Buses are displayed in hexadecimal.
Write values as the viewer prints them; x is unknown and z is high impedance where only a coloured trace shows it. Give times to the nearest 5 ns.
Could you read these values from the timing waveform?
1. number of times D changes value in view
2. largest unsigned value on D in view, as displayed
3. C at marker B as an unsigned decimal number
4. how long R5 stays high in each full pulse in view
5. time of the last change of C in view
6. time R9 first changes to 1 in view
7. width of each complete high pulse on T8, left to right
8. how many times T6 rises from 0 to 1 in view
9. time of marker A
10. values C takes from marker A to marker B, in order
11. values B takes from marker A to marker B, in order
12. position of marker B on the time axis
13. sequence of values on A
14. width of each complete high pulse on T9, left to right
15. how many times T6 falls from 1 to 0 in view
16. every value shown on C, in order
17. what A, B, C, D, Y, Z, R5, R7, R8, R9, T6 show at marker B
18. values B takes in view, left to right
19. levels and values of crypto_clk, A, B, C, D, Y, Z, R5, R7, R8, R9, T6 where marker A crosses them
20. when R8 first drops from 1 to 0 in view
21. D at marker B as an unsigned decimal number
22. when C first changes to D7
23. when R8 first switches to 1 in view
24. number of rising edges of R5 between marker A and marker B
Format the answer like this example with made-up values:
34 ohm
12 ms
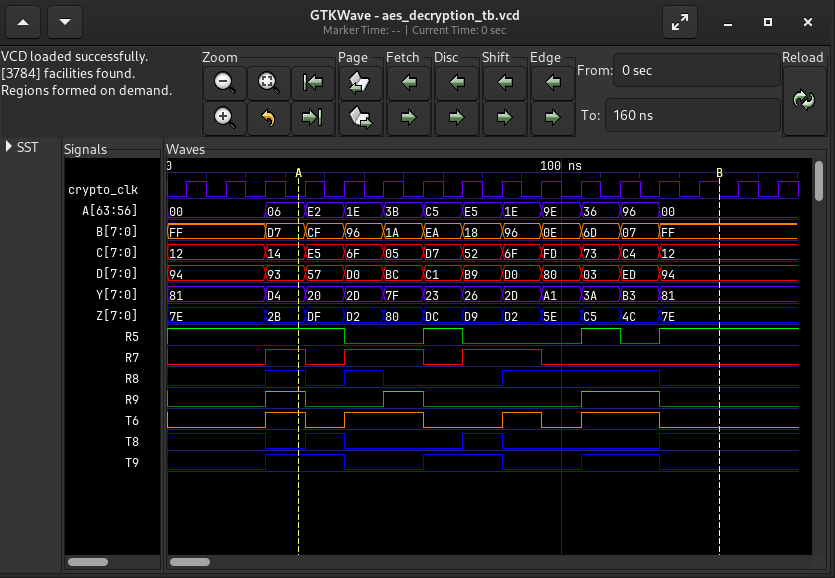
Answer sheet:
11
ED
18
10 ns, 10 ns
125 ns
25 ns
10 ns, 10 ns
4
35 ns
14, E5, 6F, 05, D7, 52, 6F, FD, 73, C4, 12
D7, CF, 96, 1A, EA, 18, 96, 0E, 6D, 07, FF
140 ns
00, 06, E2, 1E, 3B, C5, E5, 1E, 9E, 36, 96, 00
20 ns, 20 ns, 20 ns
4
12, 14, E5, 6F, 05, D7, 52, 6F, FD, 73, C4, 12
A=00, B=FF, C=12, D=94, Y=81, Z=7E, R5=1, R7=0, R8=0, R9=0, T6=0
FF, D7, CF, 96, 1A, EA, 18, 96, 0E, 6D, 07, FF
crypto_clk=0, A=06, B=D7, C=14, D=93, Y=D4, Z=2B, R5=1, R7=1, R8=1, R9=1, T6=1
35 ns
148
65 ns
25 ns
3
